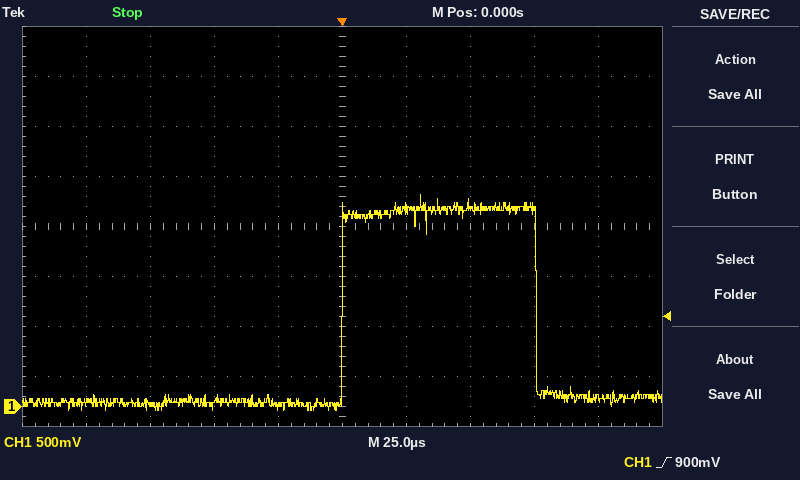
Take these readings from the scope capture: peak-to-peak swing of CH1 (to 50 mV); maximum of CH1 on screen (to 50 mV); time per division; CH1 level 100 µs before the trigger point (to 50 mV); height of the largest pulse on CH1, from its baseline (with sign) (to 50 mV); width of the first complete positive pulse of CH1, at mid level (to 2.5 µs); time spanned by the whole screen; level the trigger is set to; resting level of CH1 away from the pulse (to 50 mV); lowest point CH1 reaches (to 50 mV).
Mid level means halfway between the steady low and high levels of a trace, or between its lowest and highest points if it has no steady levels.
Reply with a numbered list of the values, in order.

1. 2.15 V
2. 2.10 V
3. 25 µs
4. 50 mV
5. +2.05 V
6. 75.0 µs
7. 250 µs
8. 900 mV
9. 50 mV
10. -50 mV
